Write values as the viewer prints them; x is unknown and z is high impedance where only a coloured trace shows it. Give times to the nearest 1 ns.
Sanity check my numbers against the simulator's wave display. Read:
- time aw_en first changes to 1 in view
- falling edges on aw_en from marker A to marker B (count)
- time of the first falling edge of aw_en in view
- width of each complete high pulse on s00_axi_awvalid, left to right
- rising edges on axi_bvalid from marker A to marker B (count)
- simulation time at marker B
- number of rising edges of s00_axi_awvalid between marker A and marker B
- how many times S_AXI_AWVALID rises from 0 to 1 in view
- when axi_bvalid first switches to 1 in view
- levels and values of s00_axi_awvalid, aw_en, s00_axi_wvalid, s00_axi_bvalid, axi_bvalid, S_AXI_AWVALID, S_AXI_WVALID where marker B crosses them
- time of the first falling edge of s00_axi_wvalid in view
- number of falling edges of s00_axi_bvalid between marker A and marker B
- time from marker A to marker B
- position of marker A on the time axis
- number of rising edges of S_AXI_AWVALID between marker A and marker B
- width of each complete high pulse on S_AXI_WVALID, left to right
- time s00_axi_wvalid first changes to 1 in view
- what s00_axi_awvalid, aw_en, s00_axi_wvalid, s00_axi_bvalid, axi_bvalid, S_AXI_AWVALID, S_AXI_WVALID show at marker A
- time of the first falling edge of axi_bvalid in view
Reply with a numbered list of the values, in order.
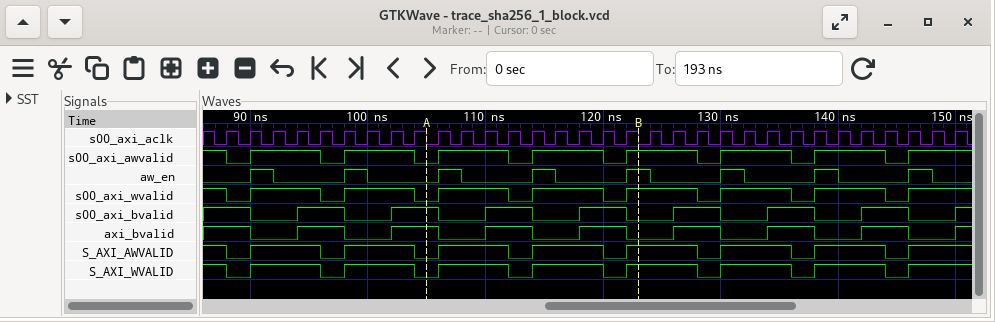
1. 90 ns
2. 2
3. 92 ns
4. 6 ns, 6 ns, 6 ns, 6 ns, 6 ns, 6 ns, 6 ns
5. 2
6. 123 ns
7. 3
8. 8
9. 94 ns
10. s00_axi_awvalid=1, aw_en=1, s00_axi_wvalid=1, s00_axi_bvalid=0, axi_bvalid=0, S_AXI_AWVALID=1, S_AXI_WVALID=1
11. 88 ns
12. 3
13. 18 ns
14. 105 ns
15. 3
16. 6 ns, 6 ns, 6 ns, 6 ns, 6 ns, 6 ns, 6 ns
17. 90 ns
18. s00_axi_awvalid=0, aw_en=0, s00_axi_wvalid=0, s00_axi_bvalid=1, axi_bvalid=1, S_AXI_AWVALID=0, S_AXI_WVALID=0
19. 90 ns
